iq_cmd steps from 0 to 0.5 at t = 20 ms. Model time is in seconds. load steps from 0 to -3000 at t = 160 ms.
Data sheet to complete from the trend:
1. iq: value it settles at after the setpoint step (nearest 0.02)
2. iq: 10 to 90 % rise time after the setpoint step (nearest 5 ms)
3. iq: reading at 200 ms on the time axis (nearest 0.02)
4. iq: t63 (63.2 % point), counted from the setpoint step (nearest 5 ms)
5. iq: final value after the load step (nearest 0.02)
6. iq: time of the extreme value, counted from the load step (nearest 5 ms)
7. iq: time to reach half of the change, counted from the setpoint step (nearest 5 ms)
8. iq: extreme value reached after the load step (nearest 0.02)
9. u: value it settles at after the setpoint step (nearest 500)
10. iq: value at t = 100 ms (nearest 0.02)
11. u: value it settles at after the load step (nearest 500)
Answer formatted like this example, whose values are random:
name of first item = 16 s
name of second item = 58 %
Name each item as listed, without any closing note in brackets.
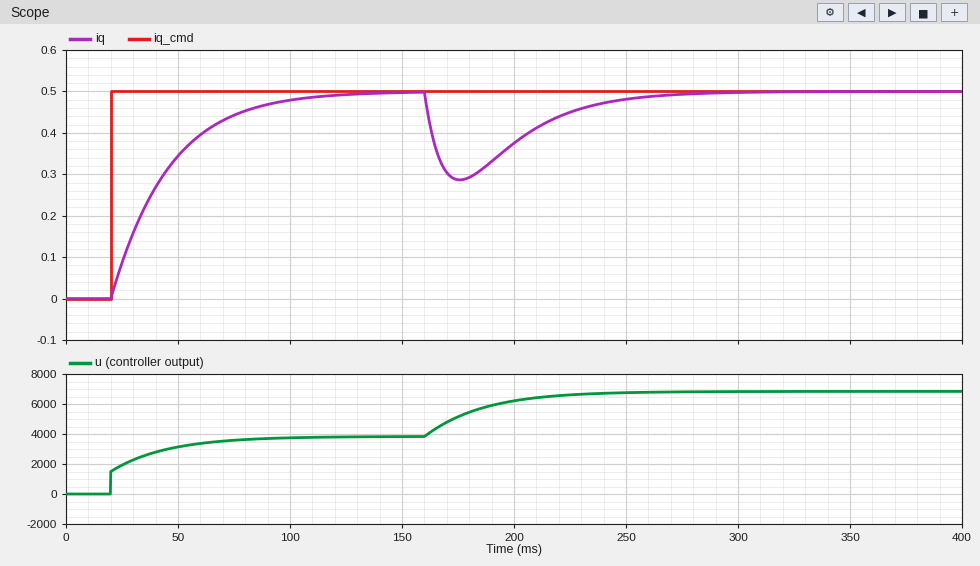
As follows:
iq: value it settles at after the setpoint step = 0.50
iq: 10 to 90 % rise time after the setpoint step = 55 ms
iq: reading at 200 ms on the time axis = 0.38
iq: t63 (63.2 % point), counted from the setpoint step = 25 ms
iq: final value after the load step = 0.50
iq: time of the extreme value, counted from the load step = 15 ms
iq: time to reach half of the change, counted from the setpoint step = 20 ms
iq: extreme value reached after the load step = 0.28
u: value it settles at after the setpoint step = 4000
iq: value at t = 100 ms = 0.48
u: value it settles at after the load step = 7000
